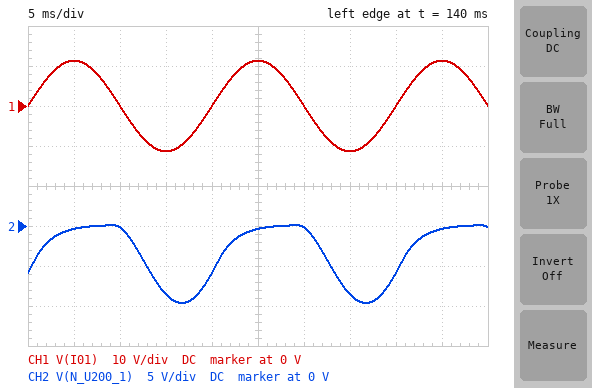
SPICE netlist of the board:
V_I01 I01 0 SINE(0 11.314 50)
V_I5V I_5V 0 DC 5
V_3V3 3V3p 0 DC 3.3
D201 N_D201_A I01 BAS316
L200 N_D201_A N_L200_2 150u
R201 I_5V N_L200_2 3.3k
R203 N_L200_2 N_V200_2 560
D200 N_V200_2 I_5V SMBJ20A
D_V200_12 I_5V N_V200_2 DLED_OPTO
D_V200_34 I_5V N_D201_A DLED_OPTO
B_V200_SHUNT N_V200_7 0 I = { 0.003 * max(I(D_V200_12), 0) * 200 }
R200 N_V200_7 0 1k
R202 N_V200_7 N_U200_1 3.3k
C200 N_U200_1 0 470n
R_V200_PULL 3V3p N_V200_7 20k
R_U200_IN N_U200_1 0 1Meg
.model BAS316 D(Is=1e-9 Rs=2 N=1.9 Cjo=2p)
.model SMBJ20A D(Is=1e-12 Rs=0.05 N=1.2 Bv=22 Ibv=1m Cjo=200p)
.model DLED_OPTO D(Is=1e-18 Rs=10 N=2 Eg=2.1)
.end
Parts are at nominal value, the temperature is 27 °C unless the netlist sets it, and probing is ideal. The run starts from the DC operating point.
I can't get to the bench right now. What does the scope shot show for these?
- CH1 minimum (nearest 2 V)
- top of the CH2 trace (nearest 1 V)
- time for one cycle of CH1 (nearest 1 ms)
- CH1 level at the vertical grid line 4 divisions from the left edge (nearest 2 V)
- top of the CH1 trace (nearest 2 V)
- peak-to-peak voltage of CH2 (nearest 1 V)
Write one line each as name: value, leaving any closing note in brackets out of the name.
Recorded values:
CH1 minimum: -12 V
top of the CH2 trace: 0 V
time for one cycle of CH1: 20 ms
CH1 level at the vertical grid line 4 divisions from the left edge: 0 V
top of the CH1 trace: 12 V
peak-to-peak voltage of CH2: 10 V
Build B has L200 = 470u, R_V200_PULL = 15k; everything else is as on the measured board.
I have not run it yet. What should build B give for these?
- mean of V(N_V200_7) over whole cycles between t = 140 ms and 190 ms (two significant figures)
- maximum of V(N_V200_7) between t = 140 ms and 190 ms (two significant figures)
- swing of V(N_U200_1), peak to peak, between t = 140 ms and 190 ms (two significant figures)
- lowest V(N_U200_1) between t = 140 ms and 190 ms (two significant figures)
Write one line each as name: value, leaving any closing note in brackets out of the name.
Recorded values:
mean of V(N_V200_7) over whole cycles between t = 140 ms and 190 ms: -3.7 V
maximum of V(N_V200_7) between t = 140 ms and 190 ms: 190 mV
swing of V(N_U200_1), peak to peak, between t = 140 ms and 190 ms: 9.6 V
lowest V(N_U200_1) between t = 140 ms and 190 ms: -9.4 V
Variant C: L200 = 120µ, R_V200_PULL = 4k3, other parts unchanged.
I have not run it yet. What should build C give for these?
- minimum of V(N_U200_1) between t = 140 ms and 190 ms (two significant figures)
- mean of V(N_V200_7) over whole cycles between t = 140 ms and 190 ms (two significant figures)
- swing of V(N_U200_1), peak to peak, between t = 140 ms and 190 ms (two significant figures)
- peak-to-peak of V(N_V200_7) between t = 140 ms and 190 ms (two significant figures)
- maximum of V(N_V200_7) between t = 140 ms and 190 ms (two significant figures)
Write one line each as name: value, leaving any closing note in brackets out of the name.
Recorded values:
minimum of V(N_U200_1) between t = 140 ms and 190 ms: -7.8 V
mean of V(N_V200_7) over whole cycles between t = 140 ms and 190 ms: -2.7 V
swing of V(N_U200_1), peak to peak, between t = 140 ms and 190 ms: 8.3 V
peak-to-peak of V(N_V200_7) between t = 140 ms and 190 ms: 9.1 V
maximum of V(N_V200_7) between t = 140 ms and 190 ms: 610 mV
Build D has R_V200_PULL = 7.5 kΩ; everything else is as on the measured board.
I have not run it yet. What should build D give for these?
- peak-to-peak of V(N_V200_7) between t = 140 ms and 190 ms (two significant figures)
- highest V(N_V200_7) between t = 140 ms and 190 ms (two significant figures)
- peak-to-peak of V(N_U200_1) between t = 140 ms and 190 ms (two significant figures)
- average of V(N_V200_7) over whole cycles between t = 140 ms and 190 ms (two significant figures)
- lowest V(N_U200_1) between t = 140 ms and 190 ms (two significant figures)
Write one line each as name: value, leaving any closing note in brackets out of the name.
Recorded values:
peak-to-peak of V(N_V200_7) between t = 140 ms and 190 ms: 9.9 V
highest V(N_V200_7) between t = 140 ms and 190 ms: 380 mV
peak-to-peak of V(N_U200_1) between t = 140 ms and 190 ms: 9.0 V
average of V(N_V200_7) over whole cycles between t = 140 ms and 190 ms: -3.3 V
lowest V(N_U200_1) between t = 140 ms and 190 ms: -8.7 V
